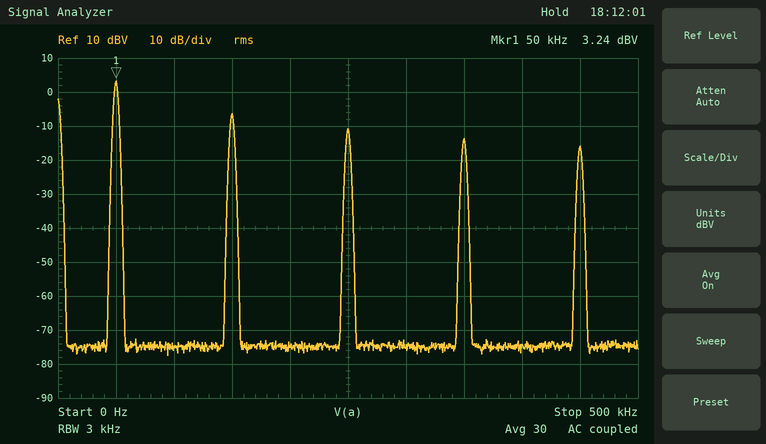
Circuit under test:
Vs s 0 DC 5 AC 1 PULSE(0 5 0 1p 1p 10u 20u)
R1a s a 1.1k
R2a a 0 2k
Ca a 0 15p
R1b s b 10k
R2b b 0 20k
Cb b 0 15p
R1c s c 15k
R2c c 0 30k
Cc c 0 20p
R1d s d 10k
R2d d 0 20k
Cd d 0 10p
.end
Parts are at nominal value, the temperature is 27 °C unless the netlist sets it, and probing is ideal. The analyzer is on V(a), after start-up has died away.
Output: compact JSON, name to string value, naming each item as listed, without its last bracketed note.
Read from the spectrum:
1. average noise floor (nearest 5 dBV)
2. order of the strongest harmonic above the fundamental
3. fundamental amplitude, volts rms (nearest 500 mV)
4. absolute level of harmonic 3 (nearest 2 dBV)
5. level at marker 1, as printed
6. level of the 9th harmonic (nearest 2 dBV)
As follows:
{"average noise floor": "-75 dBV", "order of the strongest harmonic above the fundamental": "3", "fundamental amplitude, volts rms": "1.5 V", "absolute level of harmonic 3": "-6 dBV", "level at marker 1, as printed": "3.24 dBV", "level of the 9th harmonic": "-16 dBV"}
